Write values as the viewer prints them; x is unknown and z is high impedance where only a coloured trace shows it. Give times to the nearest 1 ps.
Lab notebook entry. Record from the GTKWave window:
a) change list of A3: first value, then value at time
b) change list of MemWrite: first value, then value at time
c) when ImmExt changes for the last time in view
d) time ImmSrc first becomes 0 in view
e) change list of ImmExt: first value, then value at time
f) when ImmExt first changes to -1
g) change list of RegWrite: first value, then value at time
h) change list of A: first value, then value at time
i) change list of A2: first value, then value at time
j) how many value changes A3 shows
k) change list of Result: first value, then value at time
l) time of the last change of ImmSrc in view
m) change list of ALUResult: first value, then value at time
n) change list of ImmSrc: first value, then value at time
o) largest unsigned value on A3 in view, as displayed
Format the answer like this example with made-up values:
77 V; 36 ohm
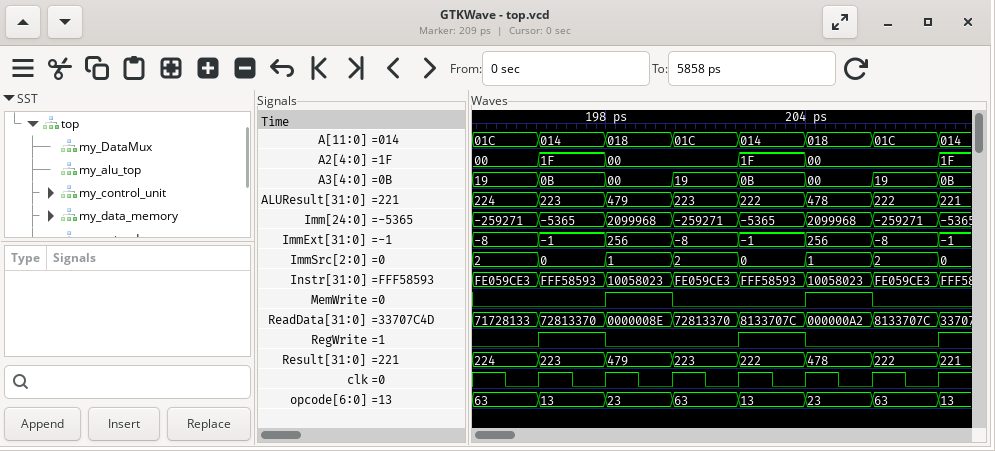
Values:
19, 0B at 196 ps, 00 at 198 ps, 19 at 200 ps, 0B at 202 ps, 00 at 204 ps, 19 at 206 ps, 0B at 208 ps; 0, 1 at 198 ps, 0 at 200 ps, 1 at 204 ps, 0 at 206 ps; 208 ps; 196 ps; -8, -1 at 196 ps, 256 at 198 ps, -8 at 200 ps, -1 at 202 ps, 256 at 204 ps, -8 at 206 ps, -1 at 208 ps; 196 ps; 0, 1 at 196 ps, 0 at 198 ps, 1 at 202 ps, 0 at 204 ps, 1 at 208 ps; 01C, 014 at 196 ps, 018 at 198 ps, 01C at 200 ps, 014 at 202 ps, 018 at 204 ps, 01C at 206 ps, 014 at 208 ps; 00, 1F at 196 ps, 00 at 198 ps, 1F at 202 ps, 00 at 204 ps, 1F at 208 ps; 7; 224, 223 at 196 ps, 479 at 198 ps, 223 at 200 ps, 222 at 202 ps, 478 at 204 ps, 222 at 206 ps, 221 at 208 ps; 208 ps; 224, 223 at 196 ps, 479 at 198 ps, 223 at 200 ps, 222 at 202 ps, 478 at 204 ps, 222 at 206 ps, 221 at 208 ps; 2, 0 at 196 ps, 1 at 198 ps, 2 at 200 ps, 0 at 202 ps, 1 at 204 ps, 2 at 206 ps, 0 at 208 ps; 19
